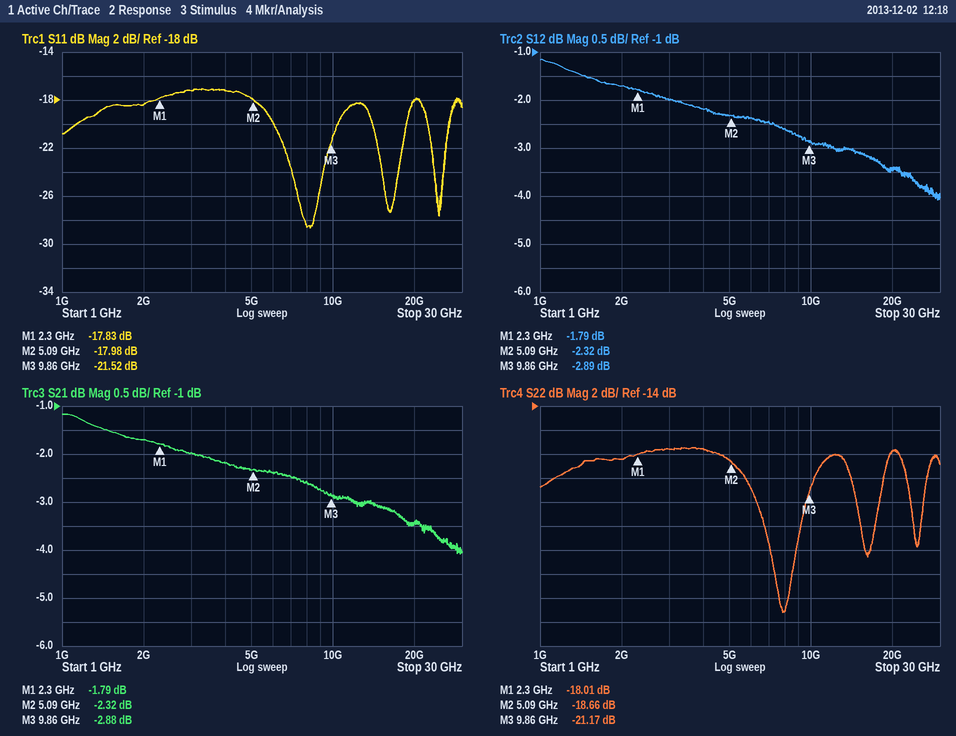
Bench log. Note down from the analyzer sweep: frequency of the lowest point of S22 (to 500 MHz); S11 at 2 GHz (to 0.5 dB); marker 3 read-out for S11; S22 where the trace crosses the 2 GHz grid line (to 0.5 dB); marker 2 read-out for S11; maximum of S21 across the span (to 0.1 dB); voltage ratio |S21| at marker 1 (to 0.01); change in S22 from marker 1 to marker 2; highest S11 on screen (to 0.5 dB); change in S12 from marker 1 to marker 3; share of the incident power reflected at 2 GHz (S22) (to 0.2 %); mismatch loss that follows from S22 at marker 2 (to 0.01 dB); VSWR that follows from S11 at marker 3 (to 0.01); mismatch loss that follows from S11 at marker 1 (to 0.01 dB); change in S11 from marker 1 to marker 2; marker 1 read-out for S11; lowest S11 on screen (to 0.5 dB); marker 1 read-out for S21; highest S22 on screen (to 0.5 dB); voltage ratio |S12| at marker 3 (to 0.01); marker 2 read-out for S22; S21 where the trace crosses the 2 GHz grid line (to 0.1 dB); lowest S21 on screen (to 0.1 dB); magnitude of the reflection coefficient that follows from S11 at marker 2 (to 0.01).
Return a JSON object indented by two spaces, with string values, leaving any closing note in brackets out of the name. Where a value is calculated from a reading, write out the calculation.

{
  "frequency of the lowest point of S22": "8.0 GHz",
  "S11 at 2 GHz": "-18.5 dB",
  "marker 3 read-out for S11": "-21.52 dB",
  "S22 where the trace crosses the 2 GHz grid line": "-18.5 dB",
  "marker 2 read-out for S11": "-17.98 dB",
  "maximum of S21 across the span": "-1.2 dB",
  "voltage ratio |S21| at marker 1": "10^(-1.79/20) ≈ 0.81",
  "change in S22 from marker 1 to marker 2": "-18.66 − (-18.01) = -0.65 dB",
  "highest S11 on screen": "-17.0 dB",
  "change in S12 from marker 1 to marker 3": "-2.89 − (-1.79) = -1.10 dB",
  "share of the incident power reflected at 2 GHz (S22)": "10^(-18.5/10) ≈ 1.4 %",
  "mismatch loss that follows from S22 at marker 2": "−10 log10(1 − 10^(-18.66/10)) ≈ 0.06 dB",
  "VSWR that follows from S11 at marker 3": "(1 + 0.0839)/(1 − 0.0839) ≈ 1.18",
  "mismatch loss that follows from S11 at marker 1": "−10 log10(1 − 10^(-17.83/10)) ≈ 0.07 dB",
  "change in S11 from marker 1 to marker 2": "-17.98 − (-17.83) = -0.15 dB",
  "marker 1 read-out for S11": "-17.83 dB",
  "lowest S11 on screen": "-28.5 dB",
  "marker 1 read-out for S21": "-1.79 dB",
  "highest S22 on screen": "-17.5 dB",
  "voltage ratio |S12| at marker 3": "10^(-2.89/20) ≈ 0.72",
  "marker 2 read-out for S22": "-18.66 dB",
  "S21 where the trace crosses the 2 GHz grid line": "-1.7 dB",
  "lowest S21 on screen": "-4.1 dB",
  "magnitude of the reflection coefficient that follows from S11 at marker 2": "10^(-17.98/20) ≈ 0.13"
}
